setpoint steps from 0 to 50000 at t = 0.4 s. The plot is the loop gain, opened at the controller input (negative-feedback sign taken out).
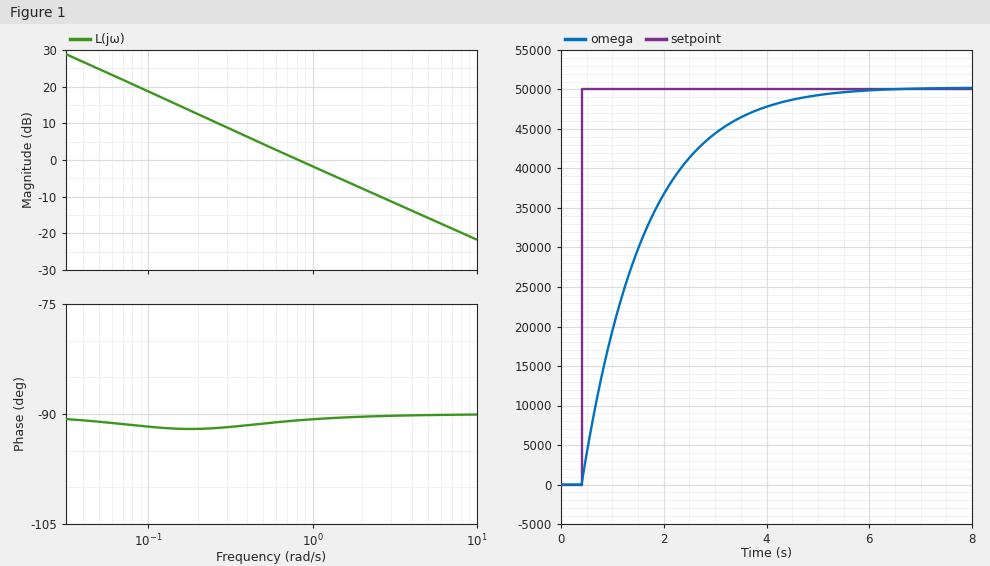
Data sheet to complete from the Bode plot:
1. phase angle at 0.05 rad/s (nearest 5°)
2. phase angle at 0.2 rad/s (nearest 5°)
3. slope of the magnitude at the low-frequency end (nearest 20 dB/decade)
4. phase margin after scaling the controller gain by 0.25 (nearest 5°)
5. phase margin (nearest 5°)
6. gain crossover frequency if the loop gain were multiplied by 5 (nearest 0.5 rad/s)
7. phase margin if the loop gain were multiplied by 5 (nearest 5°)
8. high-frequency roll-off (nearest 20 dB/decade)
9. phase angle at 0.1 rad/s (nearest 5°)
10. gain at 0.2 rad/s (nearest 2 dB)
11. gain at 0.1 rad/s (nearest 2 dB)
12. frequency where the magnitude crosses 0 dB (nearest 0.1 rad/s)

-90°
-90°
-20 dB/decade
90°
90°
4.0 rad/s
90°
-20 dB/decade
-90°
12 dB
18 dB
0.8 rad/s
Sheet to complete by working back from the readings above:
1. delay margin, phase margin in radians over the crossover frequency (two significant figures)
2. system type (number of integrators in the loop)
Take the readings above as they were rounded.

2.0 s
1
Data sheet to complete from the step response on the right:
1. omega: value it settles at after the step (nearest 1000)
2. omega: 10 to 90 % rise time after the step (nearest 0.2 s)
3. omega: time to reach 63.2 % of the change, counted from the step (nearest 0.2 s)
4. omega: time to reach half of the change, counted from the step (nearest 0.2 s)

50000
2.6 s
1.2 s
0.8 s
